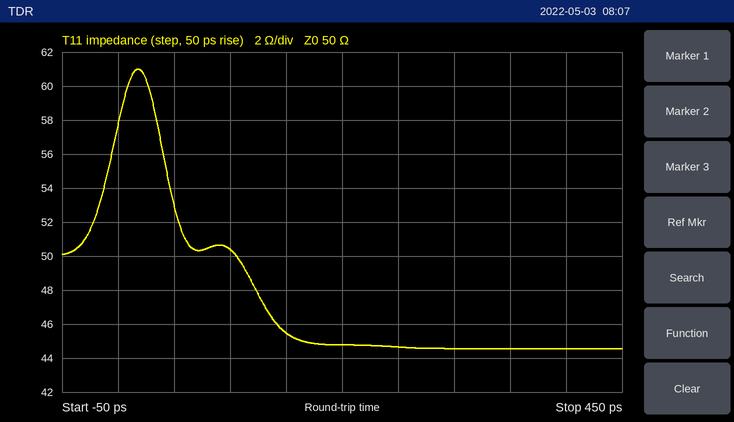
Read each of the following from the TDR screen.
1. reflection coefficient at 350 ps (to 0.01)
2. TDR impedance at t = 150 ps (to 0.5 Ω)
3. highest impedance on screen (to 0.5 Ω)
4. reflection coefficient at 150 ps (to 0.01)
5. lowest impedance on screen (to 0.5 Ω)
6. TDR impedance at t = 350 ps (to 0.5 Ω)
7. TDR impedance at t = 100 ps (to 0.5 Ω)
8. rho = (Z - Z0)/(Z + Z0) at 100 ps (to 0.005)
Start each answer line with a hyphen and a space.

- -0.06
- 45.5 Ω
- 61.0 Ω
- -0.05
- 44.5 Ω
- 44.5 Ω
- 50.5 Ω
- +0.005
